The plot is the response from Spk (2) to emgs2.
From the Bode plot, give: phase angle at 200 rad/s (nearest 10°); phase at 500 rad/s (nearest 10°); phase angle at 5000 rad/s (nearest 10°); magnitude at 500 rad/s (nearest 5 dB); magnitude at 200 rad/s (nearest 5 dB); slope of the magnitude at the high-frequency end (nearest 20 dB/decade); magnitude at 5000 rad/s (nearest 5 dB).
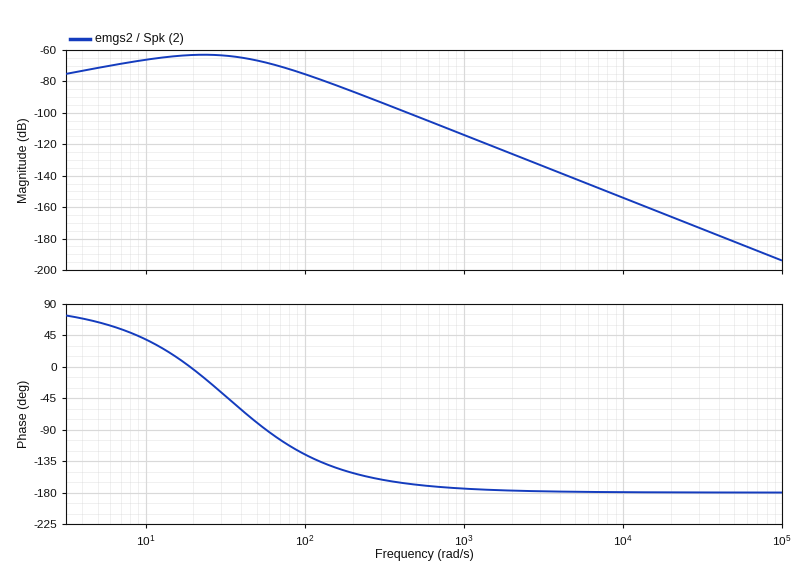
-150°
-170°
-180°
-100 dB
-85 dB
-40 dB/decade
-140 dB
